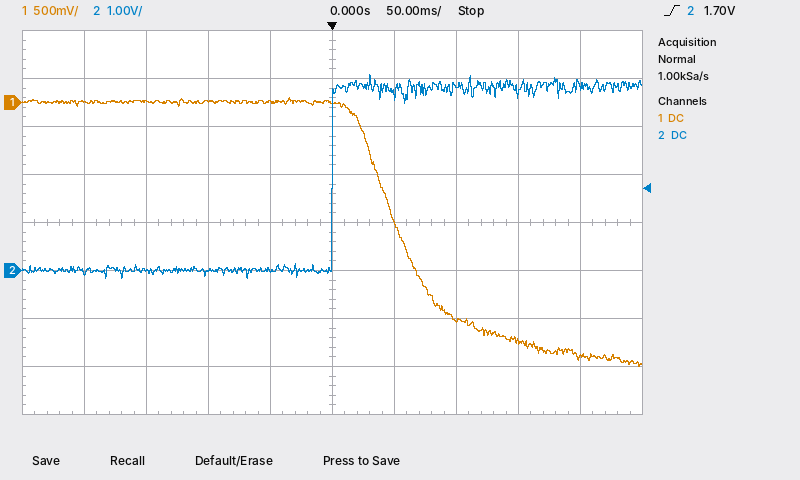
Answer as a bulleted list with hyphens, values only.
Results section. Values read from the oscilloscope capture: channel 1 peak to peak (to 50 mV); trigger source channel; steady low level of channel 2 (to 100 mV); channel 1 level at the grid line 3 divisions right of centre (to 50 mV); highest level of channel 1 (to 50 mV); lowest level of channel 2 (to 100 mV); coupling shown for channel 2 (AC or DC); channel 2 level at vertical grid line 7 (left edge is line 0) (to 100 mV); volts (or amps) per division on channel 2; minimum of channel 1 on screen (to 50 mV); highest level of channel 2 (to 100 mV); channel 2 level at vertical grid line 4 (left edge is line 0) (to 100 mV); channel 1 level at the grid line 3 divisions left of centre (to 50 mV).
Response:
- 2.80 V
- channel 2
- 0.0 V
- -2.50 V
- 50 mV
- -200 mV
- DC
- 3.9 V
- 1 V
- -2.75 V
- 4.1 V
- 0.0 V
- 0 mV
